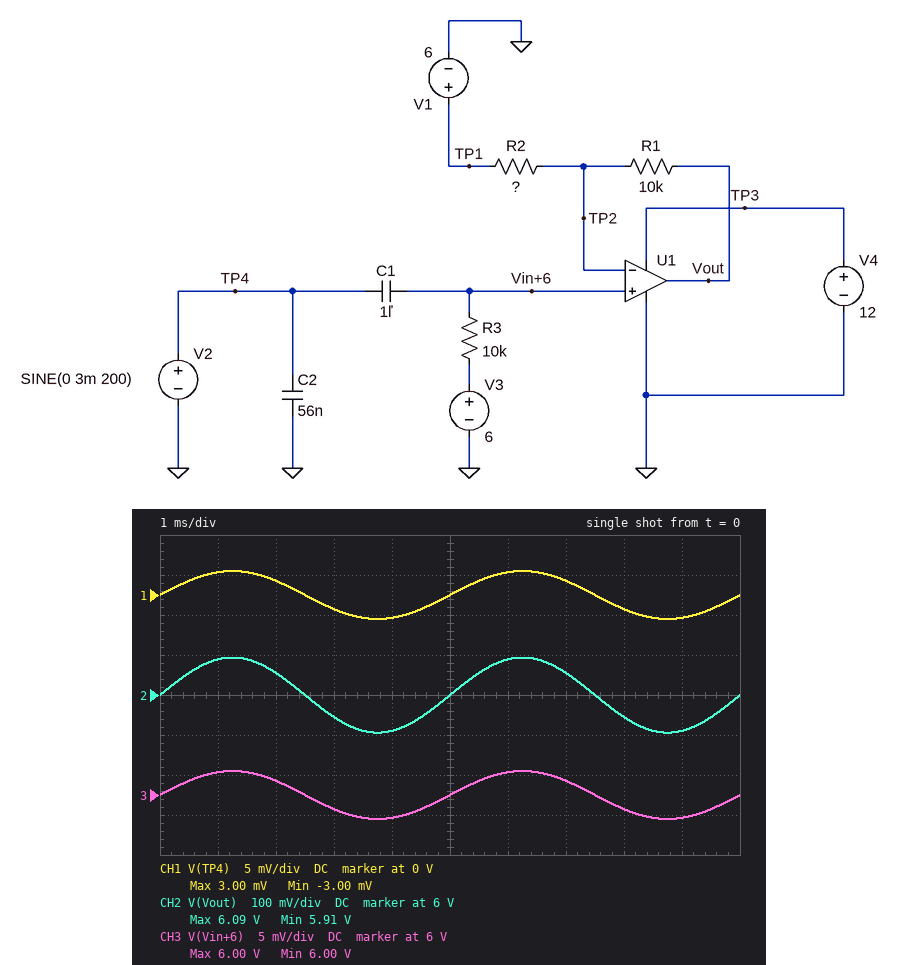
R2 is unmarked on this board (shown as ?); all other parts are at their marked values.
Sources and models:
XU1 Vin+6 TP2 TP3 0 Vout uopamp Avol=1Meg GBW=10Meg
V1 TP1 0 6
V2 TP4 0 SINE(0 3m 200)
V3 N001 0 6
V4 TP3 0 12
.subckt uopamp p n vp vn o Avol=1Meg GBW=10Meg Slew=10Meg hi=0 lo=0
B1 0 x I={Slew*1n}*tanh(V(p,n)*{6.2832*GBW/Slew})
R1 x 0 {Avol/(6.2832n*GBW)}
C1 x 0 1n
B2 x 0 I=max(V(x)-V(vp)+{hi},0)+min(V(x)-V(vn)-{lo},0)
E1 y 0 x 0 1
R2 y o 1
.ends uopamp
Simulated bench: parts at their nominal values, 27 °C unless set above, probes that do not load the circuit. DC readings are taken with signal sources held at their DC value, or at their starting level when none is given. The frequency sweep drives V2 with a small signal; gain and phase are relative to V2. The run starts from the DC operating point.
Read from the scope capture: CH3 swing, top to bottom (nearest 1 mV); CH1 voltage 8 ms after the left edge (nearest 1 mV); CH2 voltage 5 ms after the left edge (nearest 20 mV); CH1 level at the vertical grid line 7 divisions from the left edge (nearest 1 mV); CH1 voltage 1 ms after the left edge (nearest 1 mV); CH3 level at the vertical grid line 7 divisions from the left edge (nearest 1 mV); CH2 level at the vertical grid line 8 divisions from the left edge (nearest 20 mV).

6 mV
-2 mV
6.00 V
2 mV
3 mV
6.002 V
5.94 V
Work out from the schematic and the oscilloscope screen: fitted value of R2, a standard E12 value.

330 Ω
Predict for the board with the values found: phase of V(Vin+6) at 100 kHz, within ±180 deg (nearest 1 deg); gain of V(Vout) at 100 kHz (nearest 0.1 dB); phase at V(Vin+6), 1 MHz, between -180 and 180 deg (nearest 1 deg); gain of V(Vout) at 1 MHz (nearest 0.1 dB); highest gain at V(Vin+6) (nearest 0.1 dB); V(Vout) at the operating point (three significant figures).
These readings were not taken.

0 deg
29.5 dB
0 deg
19.6 dB
0 dB
6.00 V
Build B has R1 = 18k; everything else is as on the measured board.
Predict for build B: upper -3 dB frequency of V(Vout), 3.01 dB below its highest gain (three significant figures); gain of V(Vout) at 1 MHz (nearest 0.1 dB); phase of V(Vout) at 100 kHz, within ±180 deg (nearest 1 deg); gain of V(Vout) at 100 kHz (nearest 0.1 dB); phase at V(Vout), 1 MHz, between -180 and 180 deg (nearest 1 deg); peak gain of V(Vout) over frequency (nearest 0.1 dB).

180 kHz
19.9 dB
-29 deg
33.7 dB
-80 deg
34.9 dB
